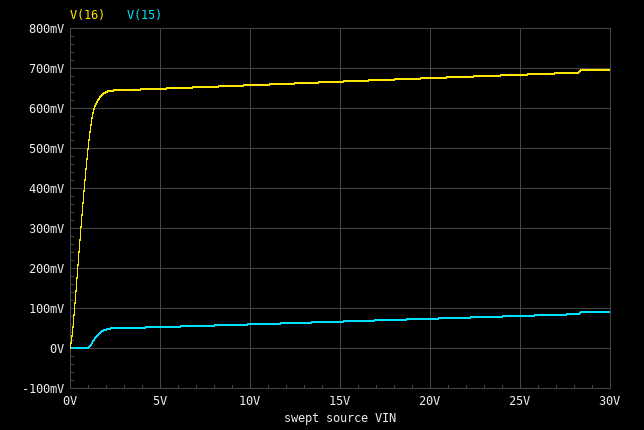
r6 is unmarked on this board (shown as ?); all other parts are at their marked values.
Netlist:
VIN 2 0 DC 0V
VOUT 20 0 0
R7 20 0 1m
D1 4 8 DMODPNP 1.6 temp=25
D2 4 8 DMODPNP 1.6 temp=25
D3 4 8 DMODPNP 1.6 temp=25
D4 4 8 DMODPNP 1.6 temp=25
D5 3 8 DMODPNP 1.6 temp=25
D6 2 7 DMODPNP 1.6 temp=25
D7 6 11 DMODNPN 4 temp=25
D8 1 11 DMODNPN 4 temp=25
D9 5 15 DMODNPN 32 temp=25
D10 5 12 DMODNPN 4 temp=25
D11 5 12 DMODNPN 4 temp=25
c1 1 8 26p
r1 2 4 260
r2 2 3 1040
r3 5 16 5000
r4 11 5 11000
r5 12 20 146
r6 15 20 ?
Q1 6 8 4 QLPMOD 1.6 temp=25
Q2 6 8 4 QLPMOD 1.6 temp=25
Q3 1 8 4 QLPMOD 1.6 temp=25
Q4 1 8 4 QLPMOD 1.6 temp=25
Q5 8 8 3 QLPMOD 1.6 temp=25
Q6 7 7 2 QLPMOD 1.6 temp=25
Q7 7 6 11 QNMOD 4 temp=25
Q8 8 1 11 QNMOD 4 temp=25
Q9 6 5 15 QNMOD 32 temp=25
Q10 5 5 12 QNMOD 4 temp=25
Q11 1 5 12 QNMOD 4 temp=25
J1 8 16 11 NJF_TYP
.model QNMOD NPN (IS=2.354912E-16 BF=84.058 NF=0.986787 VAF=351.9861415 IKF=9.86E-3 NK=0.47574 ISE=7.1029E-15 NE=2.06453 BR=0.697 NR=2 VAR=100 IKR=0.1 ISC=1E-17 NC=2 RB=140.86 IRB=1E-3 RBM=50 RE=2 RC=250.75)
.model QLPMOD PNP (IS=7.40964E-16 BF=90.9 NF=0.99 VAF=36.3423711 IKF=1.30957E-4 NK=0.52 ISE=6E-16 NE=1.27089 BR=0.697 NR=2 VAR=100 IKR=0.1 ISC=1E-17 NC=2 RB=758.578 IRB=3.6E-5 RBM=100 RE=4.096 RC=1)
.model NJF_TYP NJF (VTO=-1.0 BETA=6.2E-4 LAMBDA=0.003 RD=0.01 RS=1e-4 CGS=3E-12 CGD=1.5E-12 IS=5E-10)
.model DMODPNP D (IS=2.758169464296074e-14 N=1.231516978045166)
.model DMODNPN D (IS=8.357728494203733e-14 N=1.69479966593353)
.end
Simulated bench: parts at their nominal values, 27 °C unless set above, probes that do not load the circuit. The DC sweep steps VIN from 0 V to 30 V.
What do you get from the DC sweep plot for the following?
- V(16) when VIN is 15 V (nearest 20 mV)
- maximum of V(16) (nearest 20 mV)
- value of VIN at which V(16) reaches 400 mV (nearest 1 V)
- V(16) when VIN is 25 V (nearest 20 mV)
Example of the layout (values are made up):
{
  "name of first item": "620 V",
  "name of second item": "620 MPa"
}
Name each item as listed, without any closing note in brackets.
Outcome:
{
  "V(16) when VIN is 15 V": "660 mV",
  "maximum of V(16)": "700 mV",
  "value of VIN at which V(16) reaches 400 mV": "1 V",
  "V(16) when VIN is 25 V": "680 mV"
}
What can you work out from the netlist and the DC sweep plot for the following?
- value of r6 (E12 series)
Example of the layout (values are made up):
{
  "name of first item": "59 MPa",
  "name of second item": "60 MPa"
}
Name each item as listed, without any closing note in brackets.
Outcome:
{
  "value of r6": "680 Ω"
}
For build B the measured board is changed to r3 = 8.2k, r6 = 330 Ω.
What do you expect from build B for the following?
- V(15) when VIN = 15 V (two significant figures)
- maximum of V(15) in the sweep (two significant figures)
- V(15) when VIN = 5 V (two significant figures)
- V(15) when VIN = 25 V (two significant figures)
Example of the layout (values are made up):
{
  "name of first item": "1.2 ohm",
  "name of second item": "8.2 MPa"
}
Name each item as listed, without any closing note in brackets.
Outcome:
{
  "V(15) when VIN = 15 V": "100 mV",
  "maximum of V(15) in the sweep": "150 mV",
  "V(15) when VIN = 5 V": "76 mV",
  "V(15) when VIN = 25 V": "130 mV"
}
